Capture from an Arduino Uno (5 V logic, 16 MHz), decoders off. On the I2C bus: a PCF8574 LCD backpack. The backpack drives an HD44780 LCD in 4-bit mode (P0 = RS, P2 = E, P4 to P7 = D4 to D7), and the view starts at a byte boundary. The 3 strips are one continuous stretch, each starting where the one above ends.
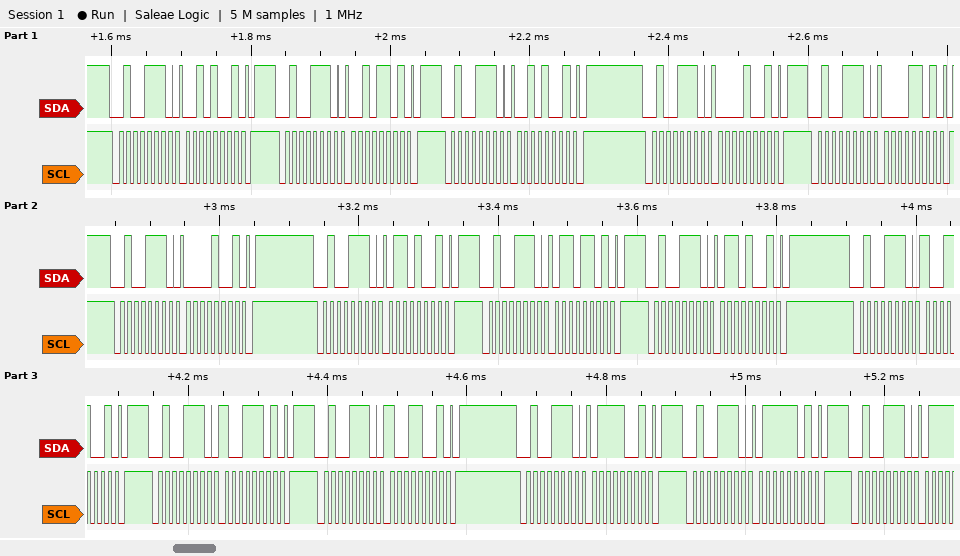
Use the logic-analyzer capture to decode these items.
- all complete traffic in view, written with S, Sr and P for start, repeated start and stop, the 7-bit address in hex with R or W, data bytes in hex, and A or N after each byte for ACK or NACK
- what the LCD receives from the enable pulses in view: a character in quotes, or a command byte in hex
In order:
S 27W A 29 A P S 27W A 2D A P S 27W A 29 A P S 27W A 09 A P S 27W A 0D A P S 27W A 09 A P S 27W A 69 A P S 27W A 6D A P S 27W A 69 A P S 27W A 99 A P S 27W A 9D A P S 27W A 99 A P S 27W A 79 A P S 27W A 7D A P S 27W A
' ' 'i'
